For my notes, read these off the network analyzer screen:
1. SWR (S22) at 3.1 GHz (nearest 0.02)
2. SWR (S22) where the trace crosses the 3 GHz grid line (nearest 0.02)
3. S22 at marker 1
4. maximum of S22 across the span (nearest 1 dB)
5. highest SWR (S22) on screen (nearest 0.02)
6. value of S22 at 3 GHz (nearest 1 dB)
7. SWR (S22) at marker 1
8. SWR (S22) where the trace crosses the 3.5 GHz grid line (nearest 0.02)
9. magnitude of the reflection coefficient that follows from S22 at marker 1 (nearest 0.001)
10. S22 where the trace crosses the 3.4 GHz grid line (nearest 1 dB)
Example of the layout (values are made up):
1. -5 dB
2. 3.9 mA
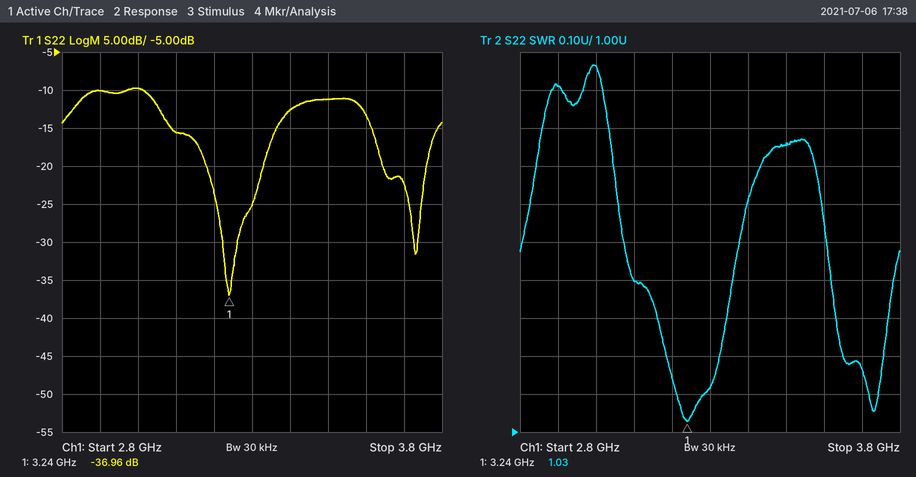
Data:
1. 1.40
2. 1.96
3. -36.96 dB
4. -10 dB
5. 1.96
6. -10 dB
7. 1.03
8. 1.76
9. 0.014
10. -13 dB
